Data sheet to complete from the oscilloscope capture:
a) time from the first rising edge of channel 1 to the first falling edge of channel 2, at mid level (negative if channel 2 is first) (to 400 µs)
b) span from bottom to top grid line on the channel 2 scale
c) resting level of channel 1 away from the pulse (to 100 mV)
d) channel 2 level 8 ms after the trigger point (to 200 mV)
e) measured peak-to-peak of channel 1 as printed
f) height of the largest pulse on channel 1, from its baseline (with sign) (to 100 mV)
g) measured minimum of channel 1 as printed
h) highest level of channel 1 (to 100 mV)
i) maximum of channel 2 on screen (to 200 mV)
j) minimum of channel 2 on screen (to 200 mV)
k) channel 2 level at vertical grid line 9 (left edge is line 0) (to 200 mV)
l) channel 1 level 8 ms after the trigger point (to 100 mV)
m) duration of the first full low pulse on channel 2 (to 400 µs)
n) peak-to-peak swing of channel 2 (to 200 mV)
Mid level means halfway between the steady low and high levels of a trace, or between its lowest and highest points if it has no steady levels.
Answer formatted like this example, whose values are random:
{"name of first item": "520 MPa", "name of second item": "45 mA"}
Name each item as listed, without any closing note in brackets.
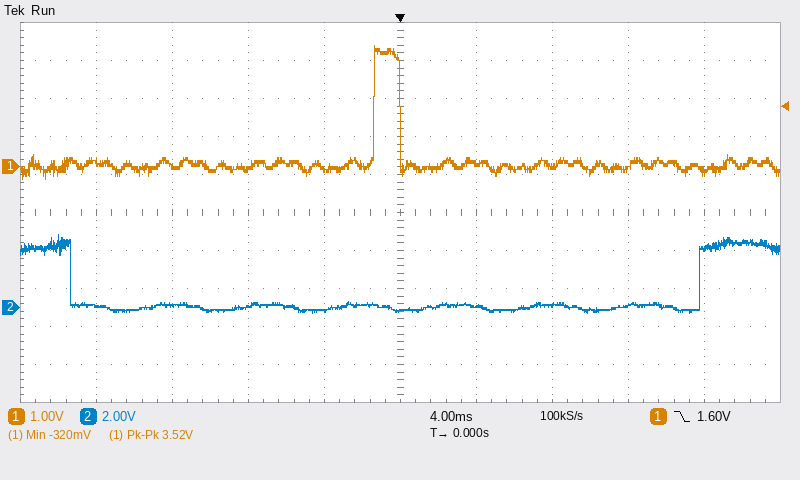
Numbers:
{"time from the first rising edge of channel 1 to the first falling edge of channel 2, at mid level (negative if channel 2 is first)": "-16.0 ms", "span from bottom to top grid line on the channel 2 scale": "20 V", "resting level of channel 1 away from the pulse": "0.0 V", "channel 2 level 8 ms after the trigger point": "200 mV", "measured peak-to-peak of channel 1 as printed": "3.52 V", "height of the largest pulse on channel 1, from its baseline (with sign)": "+3.2 V", "measured minimum of channel 1 as printed": "-320 mV", "highest level of channel 1": "3.2 V", "maximum of channel 2 on screen": "3.8 V", "minimum of channel 2 on screen": "-400 mV", "channel 2 level at vertical grid line 9 (left edge is line 0)": "3.2 V", "channel 1 level 8 ms after the trigger point": "0.0 V", "duration of the first full low pulse on channel 2": "33.2 ms", "peak-to-peak swing of channel 2": "4.2 V"}
